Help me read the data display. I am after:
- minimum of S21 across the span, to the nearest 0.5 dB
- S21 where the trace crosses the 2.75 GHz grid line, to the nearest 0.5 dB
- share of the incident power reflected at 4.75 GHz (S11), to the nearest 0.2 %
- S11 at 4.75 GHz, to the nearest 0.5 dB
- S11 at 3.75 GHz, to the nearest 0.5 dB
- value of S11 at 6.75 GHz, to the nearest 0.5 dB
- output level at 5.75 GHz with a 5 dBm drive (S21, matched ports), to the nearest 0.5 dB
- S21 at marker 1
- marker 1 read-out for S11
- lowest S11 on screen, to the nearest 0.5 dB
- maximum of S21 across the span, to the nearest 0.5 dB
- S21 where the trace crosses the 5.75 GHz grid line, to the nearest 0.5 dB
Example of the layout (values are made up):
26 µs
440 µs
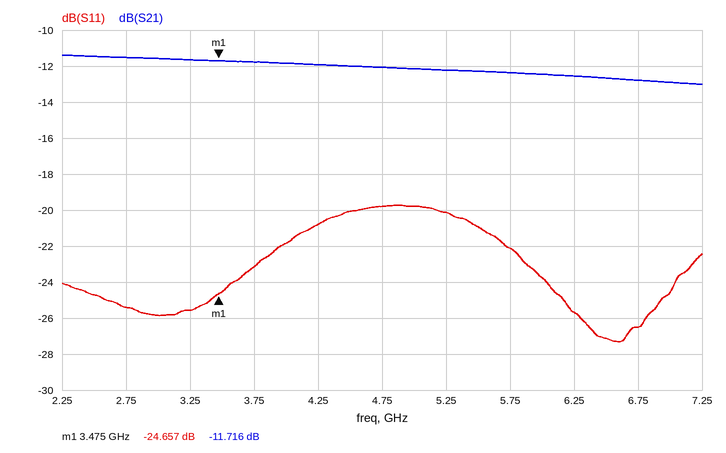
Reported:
-13.0 dB
-11.5 dB
1.0 %
-20.0 dB
-23.0 dB
-26.5 dB
-7.5 dBm
-11.716 dB
-24.657 dB
-27.5 dB
-11.5 dB
-12.5 dB
